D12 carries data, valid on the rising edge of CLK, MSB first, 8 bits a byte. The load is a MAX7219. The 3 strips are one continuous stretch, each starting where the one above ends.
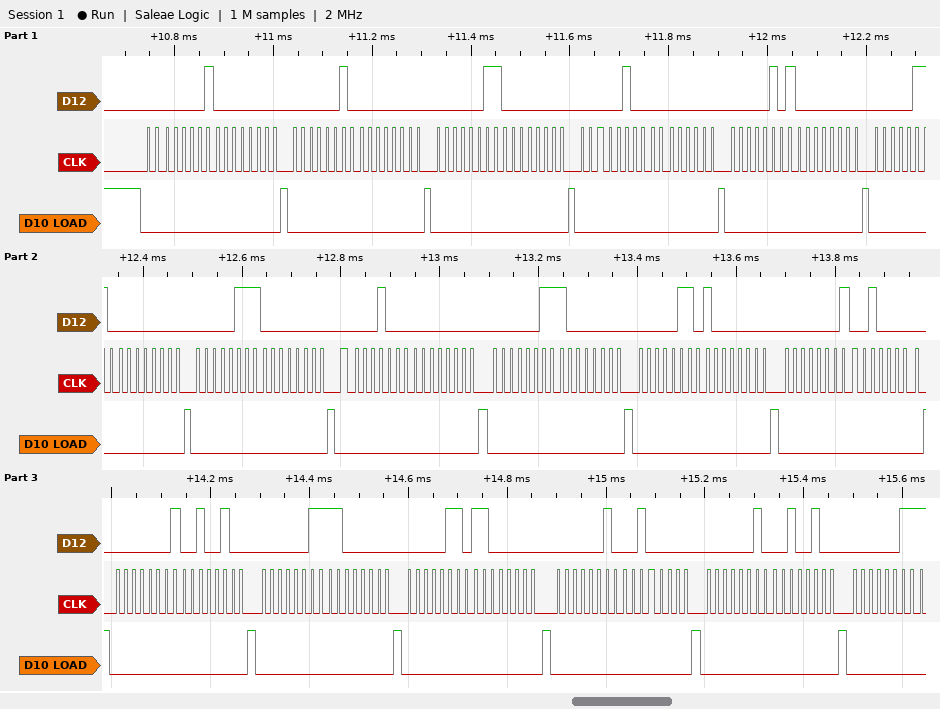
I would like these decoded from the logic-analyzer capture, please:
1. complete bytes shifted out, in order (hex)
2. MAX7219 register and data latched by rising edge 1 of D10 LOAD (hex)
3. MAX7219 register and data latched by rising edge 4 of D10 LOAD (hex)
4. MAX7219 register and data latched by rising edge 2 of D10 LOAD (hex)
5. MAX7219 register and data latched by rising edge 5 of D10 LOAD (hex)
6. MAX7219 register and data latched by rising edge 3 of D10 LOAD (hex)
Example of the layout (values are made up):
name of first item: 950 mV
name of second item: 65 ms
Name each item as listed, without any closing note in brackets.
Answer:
complete bytes shifted out, in order: 0x01 0x00 0x02 0x00 0x03 0x00 0x04 0x00 0x05 0x00 0x06 0x00 0x07 0x00 0x08 0x00 0x03 0x80 0x06 0x80 0x01 0x20 0x01 0x24 0x03 0xC0 0x06 0xC0 0x02 0x20 0x02 0x24 0x03
MAX7219 register and data latched by rising edge 1 of D10 LOAD: register 0x1, data 0x00
MAX7219 register and data latched by rising edge 4 of D10 LOAD: register 0x4, data 0x00
MAX7219 register and data latched by rising edge 2 of D10 LOAD: register 0x2, data 0x00
MAX7219 register and data latched by rising edge 5 of D10 LOAD: register 0x5, data 0x00
MAX7219 register and data latched by rising edge 3 of D10 LOAD: register 0x3, data 0x00
